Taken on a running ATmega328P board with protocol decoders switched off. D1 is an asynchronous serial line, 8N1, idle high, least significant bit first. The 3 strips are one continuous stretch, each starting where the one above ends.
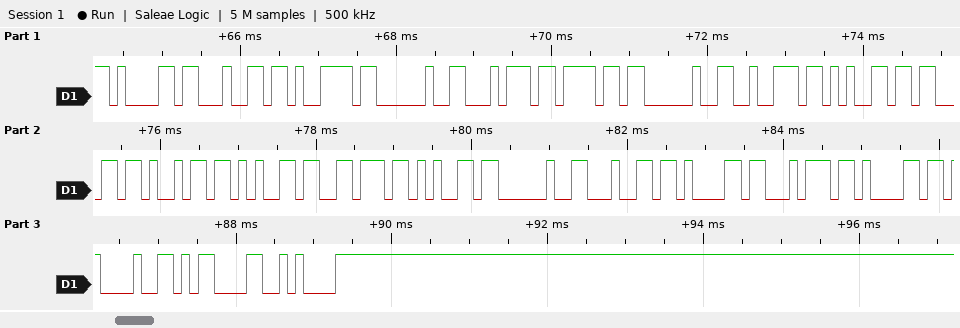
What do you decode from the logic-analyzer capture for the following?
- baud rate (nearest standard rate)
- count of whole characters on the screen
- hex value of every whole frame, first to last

9600 baud
22
61 64 79 20 74 6F 20 72 65 63 69 65 76 65 20 64 61 74 61 21 0D 0A
